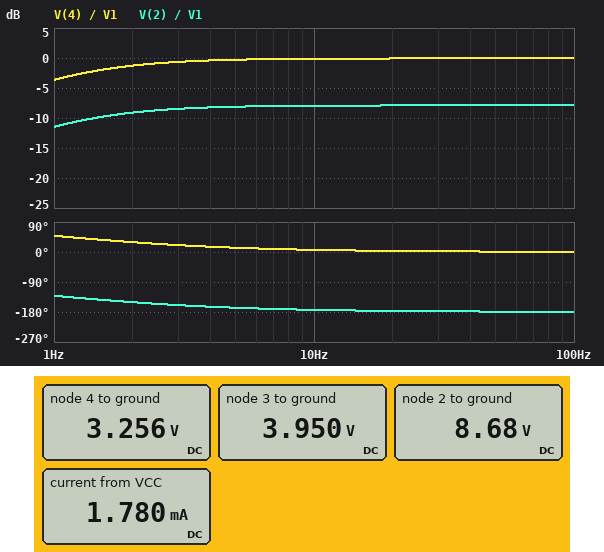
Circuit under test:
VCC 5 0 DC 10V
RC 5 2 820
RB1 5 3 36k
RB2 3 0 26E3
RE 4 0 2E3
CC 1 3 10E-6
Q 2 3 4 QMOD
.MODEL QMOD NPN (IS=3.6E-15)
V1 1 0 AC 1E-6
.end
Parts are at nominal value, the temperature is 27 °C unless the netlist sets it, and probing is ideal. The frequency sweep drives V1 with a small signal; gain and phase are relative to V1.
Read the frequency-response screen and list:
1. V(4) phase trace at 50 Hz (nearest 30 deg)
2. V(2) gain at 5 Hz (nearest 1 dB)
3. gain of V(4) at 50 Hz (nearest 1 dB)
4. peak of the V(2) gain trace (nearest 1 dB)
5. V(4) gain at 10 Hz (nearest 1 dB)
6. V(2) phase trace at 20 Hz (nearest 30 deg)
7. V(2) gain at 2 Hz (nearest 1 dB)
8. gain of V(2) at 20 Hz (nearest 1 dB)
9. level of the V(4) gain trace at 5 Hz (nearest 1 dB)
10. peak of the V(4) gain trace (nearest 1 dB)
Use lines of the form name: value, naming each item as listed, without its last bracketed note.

V(4) phase trace at 50 Hz: 0 deg
V(2) gain at 5 Hz: -8 dB
gain of V(4) at 50 Hz: 0 dB
peak of the V(2) gain trace: -8 dB
V(4) gain at 10 Hz: 0 dB
V(2) phase trace at 20 Hz: -180 deg
V(2) gain at 2 Hz: -9 dB
gain of V(2) at 20 Hz: -8 dB
level of the V(4) gain trace at 5 Hz: 0 dB
peak of the V(4) gain trace: 0 dB
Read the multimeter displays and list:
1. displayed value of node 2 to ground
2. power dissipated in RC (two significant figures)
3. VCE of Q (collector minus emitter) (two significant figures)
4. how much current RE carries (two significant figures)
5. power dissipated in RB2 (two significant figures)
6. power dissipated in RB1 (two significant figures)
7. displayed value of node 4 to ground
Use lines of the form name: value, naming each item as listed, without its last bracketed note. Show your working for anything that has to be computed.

displayed value of node 2 to ground: 8.68 V
power dissipated in RC: (10 V - 8.68 V)^2 / 820 Ω = 2.1 mW
VCE of Q (collector minus emitter): 8.68 V - 3.256 V = 5.4 V
how much current RE carries: (3.256 V) / 2 kΩ = 1.6 mA
power dissipated in RB2: (3.95 V)^2 / 26 kΩ = 600 µW
power dissipated in RB1: (10 V - 3.95 V)^2 / 36 kΩ = 1.0 mW
displayed value of node 4 to ground: 3.256 V
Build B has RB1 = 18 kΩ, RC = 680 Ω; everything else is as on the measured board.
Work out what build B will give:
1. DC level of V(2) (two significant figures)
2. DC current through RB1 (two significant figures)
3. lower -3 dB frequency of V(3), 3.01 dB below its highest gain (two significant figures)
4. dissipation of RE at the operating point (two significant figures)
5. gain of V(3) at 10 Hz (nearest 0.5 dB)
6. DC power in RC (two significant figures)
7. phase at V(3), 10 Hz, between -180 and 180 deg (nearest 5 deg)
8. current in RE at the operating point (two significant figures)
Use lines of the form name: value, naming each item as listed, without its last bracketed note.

DC level of V(2): 8.3 V
DC current through RB1: 240 µA
lower -3 dB frequency of V(3), 3.01 dB below its highest gain: 1.6 Hz
dissipation of RE at the operating point: 12 mW
gain of V(3) at 10 Hz: 0 dB
DC power in RC: 4.1 mW
phase at V(3), 10 Hz, between -180 and 180 deg: 10 deg
current in RE at the operating point: 2.5 mA
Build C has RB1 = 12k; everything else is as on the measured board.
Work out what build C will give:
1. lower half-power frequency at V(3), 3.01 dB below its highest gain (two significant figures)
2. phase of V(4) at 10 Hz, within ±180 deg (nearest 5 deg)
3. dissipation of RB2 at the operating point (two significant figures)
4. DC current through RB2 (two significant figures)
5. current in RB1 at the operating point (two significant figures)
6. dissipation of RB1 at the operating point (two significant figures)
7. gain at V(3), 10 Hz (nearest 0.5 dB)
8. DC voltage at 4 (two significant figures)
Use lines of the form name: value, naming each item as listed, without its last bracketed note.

lower half-power frequency at V(3), 3.01 dB below its highest gain: 2.0 Hz
phase of V(4) at 10 Hz, within ±180 deg: 10 deg
dissipation of RB2 at the operating point: 1.7 mW
DC current through RB2: 250 µA
current in RB1 at the operating point: 280 µA
dissipation of RB1 at the operating point: 960 µW
gain at V(3), 10 Hz: 0 dB
DC voltage at 4: 5.9 V
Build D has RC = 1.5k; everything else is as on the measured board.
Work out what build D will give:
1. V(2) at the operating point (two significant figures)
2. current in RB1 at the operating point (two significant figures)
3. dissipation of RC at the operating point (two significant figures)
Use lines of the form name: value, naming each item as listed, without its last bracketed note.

V(2) at the operating point: 7.6 V
current in RB1 at the operating point: 170 µA
dissipation of RC at the operating point: 3.9 mW
